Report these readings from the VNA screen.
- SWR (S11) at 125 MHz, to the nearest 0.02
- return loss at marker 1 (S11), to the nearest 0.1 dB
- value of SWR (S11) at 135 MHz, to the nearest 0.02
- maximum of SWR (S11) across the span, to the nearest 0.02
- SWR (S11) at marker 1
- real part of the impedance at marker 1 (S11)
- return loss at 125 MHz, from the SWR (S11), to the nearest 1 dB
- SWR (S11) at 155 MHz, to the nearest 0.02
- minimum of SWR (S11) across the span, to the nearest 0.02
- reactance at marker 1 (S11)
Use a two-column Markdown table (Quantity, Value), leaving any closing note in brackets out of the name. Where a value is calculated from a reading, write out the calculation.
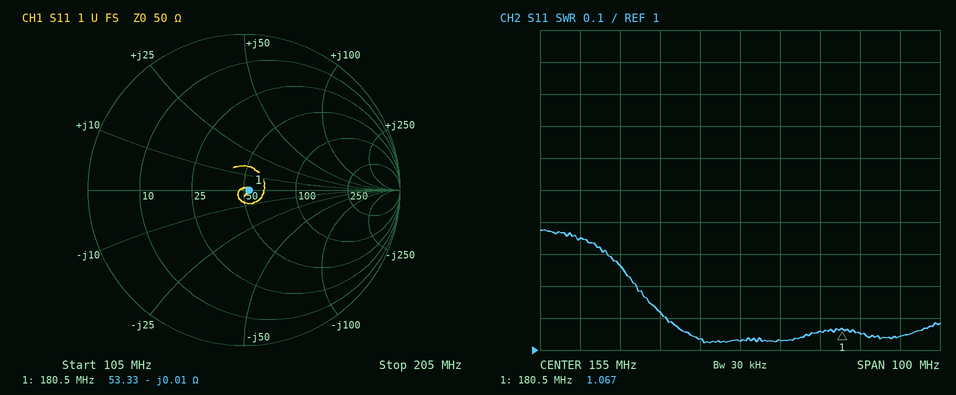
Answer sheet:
| Quantity | Value |
|---|---|
| SWR (S11) at 125 MHz, to the nearest 0.02 | 1.26 |
| return loss at marker 1 (S11), to the nearest 0.1 dB | 29.8 dB |
| value of SWR (S11) at 135 MHz, to the nearest 0.02 | 1.12 |
| maximum of SWR (S11) across the span, to the nearest 0.02 | 1.38 |
| SWR (S11) at marker 1 | 1.067 |
| real part of the impedance at marker 1 | 53.33 Ω |
| return loss at 125 MHz, from the SWR (S11), to the nearest 1 dB | −20 log10((1.26 − 1)/(1.26 + 1)) ≈ 19 dB |
| SWR (S11) at 155 MHz, to the nearest 0.02 | 1.02 |
| minimum of SWR (S11) across the span, to the nearest 0.02 | 1.02 |
| reactance at marker 1 | -0.01 Ω |
